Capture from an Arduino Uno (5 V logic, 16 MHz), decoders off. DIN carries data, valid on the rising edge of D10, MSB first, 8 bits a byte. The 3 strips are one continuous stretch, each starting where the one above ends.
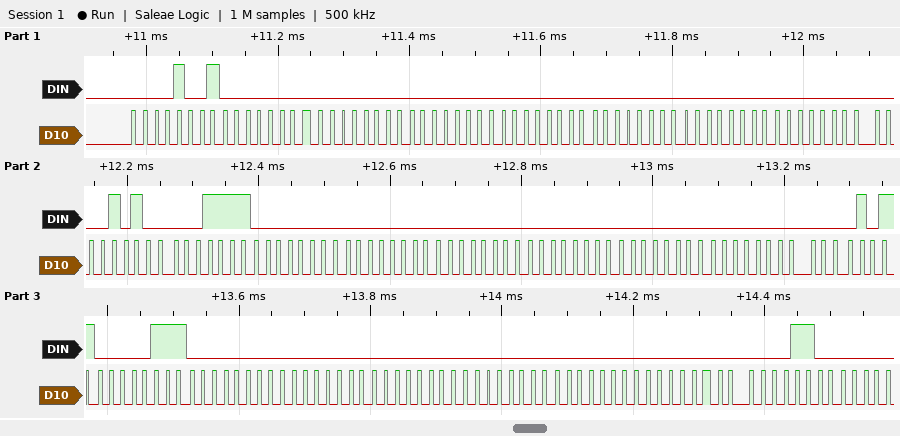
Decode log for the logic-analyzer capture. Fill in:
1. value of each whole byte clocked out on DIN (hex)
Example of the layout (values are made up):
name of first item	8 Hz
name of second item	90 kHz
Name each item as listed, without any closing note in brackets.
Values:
value of each whole byte clocked out on DIN	09 00 00 00 00 00 00 00 0A 0F 00 00 00 00 00 00 0B 07 00 00 00 00 00 00 0C
